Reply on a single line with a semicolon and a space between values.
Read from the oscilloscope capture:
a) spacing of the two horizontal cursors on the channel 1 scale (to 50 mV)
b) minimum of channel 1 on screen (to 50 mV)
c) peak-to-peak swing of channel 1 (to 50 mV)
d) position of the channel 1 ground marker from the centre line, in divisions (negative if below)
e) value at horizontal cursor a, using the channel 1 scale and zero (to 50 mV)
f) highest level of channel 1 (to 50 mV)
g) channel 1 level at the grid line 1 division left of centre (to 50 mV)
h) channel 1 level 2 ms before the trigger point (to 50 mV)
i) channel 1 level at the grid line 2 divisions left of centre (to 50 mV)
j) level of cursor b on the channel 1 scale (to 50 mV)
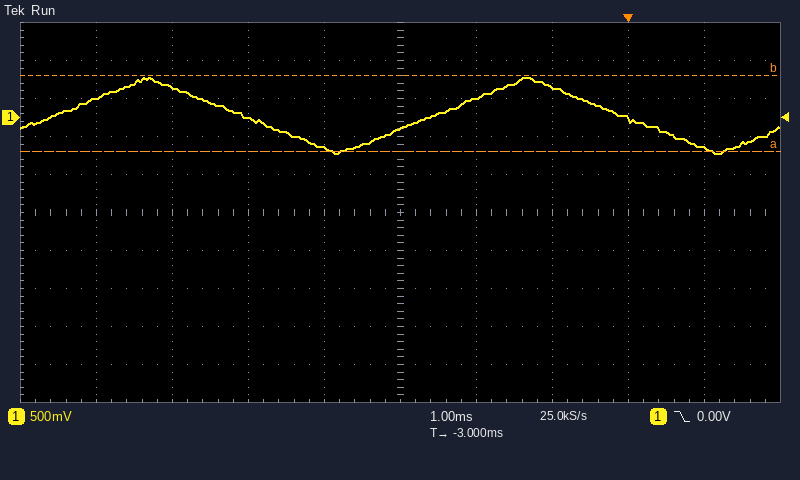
1.00 V; -450 mV; 1.00 V; +2.5 div; -450 mV; 550 mV; -400 mV; 250 mV; 0 mV; 550 mV
